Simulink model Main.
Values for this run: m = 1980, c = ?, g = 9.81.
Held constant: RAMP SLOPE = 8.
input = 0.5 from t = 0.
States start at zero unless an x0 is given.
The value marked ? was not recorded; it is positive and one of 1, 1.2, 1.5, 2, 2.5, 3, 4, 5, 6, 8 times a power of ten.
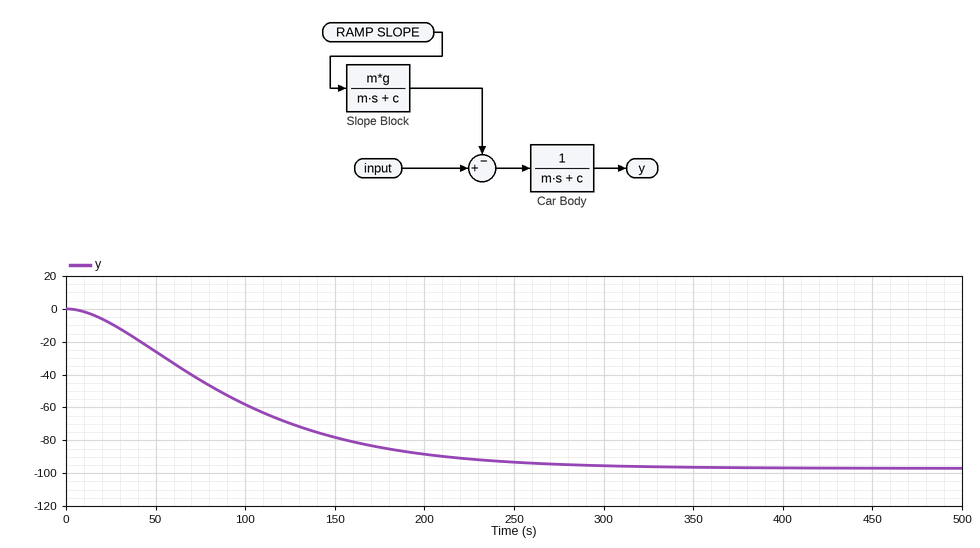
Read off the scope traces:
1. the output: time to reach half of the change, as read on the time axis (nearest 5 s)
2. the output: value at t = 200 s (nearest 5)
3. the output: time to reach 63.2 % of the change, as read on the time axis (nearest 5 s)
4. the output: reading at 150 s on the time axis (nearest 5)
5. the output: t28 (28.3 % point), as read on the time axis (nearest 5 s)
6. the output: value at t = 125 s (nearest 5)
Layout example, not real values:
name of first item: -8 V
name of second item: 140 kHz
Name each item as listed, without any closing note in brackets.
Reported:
the output: time to reach half of the change, as read on the time axis: 85 s
the output: value at t = 200 s: -90
the output: time to reach 63.2 % of the change, as read on the time axis: 105 s
the output: reading at 150 s on the time axis: -80
the output: t28 (28.3 % point), as read on the time axis: 50 s
the output: value at t = 125 s: -70
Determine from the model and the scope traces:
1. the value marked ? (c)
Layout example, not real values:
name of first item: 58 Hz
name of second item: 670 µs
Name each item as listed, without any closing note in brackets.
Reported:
the value marked ?: 40
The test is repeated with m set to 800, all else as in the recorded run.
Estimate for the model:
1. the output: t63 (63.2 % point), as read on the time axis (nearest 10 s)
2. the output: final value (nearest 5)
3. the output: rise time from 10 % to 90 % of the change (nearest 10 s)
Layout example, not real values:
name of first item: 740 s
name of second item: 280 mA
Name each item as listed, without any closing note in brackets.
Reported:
the output: t63 (63.2 % point), as read on the time axis: 40 s
the output: final value: -40
the output: rise time from 10 % to 90 % of the change: 70 s
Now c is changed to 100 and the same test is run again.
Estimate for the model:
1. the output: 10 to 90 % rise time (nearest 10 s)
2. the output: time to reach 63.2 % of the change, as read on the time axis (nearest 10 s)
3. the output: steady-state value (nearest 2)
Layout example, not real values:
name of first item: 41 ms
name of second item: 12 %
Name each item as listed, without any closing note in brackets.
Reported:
the output: 10 to 90 % rise time: 70 s
the output: time to reach 63.2 % of the change, as read on the time axis: 40 s
the output: steady-state value: -16
